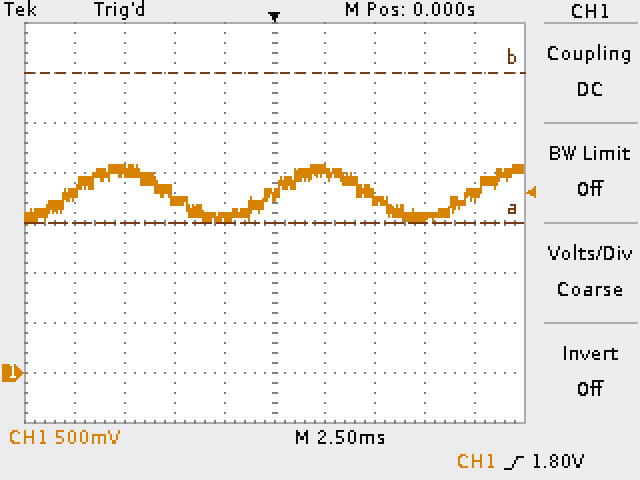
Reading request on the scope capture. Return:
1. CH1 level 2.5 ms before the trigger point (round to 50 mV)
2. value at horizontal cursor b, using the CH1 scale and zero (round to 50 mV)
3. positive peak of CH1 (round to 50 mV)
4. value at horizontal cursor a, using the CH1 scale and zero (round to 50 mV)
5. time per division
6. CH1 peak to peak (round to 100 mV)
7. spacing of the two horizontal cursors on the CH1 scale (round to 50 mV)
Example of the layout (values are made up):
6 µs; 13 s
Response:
1.55 V; 3.00 V; 2.10 V; 1.50 V; 2.5 ms; 600 mV; 1.50 V
